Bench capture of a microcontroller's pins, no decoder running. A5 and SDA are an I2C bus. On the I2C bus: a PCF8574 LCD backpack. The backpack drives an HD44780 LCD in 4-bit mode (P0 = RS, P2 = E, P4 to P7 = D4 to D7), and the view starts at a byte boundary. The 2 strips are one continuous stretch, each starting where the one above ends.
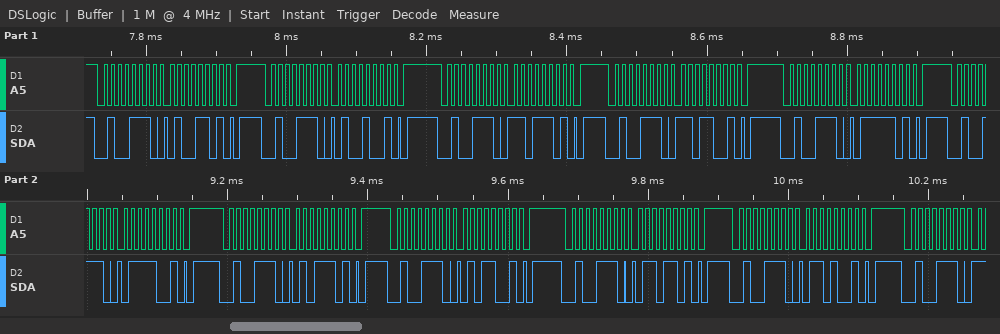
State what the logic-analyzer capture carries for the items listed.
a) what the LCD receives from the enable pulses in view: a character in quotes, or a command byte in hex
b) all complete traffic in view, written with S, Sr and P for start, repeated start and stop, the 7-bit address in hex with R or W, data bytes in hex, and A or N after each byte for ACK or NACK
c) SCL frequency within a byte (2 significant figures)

'M' 'u'
S 27W A 4D A P S 27W A 49 A P S 27W A DD A P S 27W A D9 A P S 27W A 7D A P S 27W A 79 A P S 27W A 5D A P S 27W A 59 A P S 27W A 6D A P S 27W A 69 A P S 27W A
100 kHz
